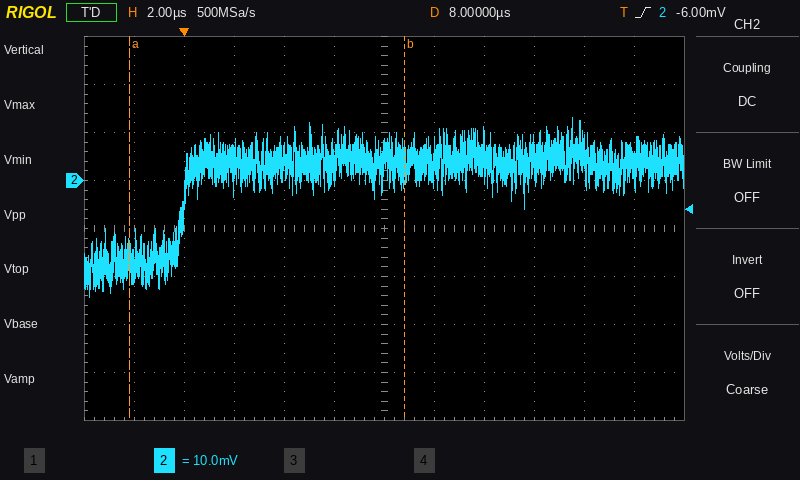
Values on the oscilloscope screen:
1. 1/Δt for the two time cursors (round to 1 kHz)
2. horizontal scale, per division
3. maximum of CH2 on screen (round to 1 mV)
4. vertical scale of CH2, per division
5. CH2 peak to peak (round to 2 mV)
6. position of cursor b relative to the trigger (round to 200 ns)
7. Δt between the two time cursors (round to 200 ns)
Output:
91 kHz
2 µs
13 mV
10 mV
38 mV
+8.8 µs
11.0 µs
